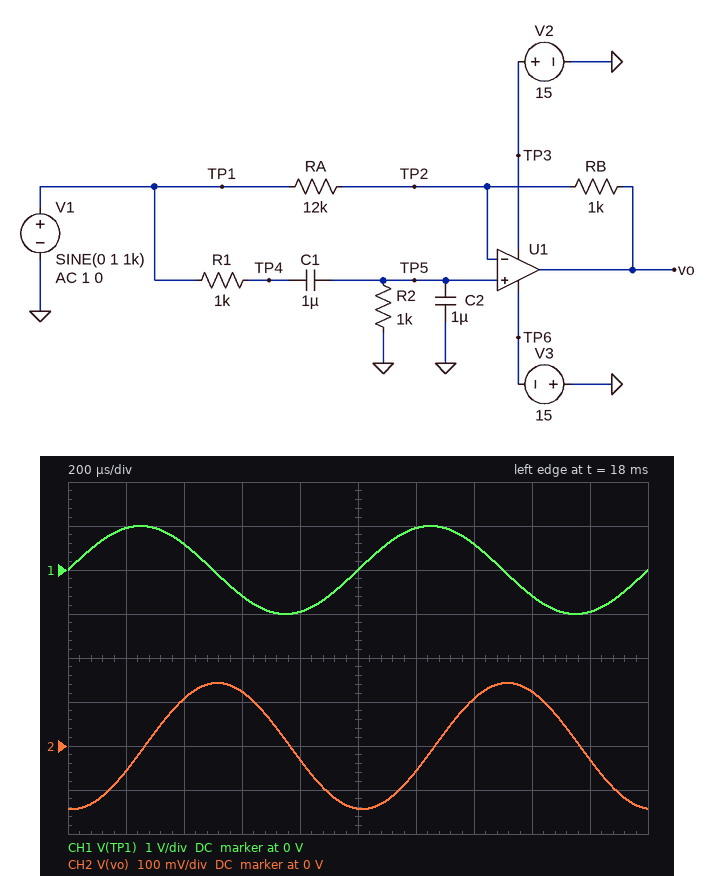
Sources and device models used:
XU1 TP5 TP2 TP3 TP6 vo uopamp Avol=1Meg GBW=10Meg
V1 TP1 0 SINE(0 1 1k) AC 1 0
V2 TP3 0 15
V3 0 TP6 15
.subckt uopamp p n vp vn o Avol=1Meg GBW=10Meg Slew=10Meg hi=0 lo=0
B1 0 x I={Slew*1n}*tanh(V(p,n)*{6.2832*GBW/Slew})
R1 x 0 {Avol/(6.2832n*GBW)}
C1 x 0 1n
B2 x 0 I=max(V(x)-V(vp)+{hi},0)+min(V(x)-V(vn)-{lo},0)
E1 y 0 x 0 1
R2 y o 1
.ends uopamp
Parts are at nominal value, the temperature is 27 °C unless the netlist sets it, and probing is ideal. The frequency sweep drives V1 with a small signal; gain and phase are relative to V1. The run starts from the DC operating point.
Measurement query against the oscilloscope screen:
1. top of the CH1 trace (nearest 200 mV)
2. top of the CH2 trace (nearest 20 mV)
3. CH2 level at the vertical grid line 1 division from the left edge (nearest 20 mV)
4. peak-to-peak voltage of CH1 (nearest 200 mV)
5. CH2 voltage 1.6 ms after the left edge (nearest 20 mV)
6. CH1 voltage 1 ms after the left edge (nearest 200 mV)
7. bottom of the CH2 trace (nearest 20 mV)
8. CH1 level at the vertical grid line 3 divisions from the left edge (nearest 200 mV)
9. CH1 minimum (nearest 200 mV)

1.0 V
140 mV
-60 mV
2.0 V
120 mV
0 V
-140 mV
-600 mV
-1.0 V
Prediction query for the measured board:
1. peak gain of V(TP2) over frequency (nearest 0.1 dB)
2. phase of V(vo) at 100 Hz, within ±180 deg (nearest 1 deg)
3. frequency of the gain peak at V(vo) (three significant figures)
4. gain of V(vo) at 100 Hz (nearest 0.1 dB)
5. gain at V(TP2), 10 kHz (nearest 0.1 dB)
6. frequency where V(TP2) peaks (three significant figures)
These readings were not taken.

-9.5 dB
23 deg
159 Hz
-11.5 dB
-36.0 dB
159 Hz
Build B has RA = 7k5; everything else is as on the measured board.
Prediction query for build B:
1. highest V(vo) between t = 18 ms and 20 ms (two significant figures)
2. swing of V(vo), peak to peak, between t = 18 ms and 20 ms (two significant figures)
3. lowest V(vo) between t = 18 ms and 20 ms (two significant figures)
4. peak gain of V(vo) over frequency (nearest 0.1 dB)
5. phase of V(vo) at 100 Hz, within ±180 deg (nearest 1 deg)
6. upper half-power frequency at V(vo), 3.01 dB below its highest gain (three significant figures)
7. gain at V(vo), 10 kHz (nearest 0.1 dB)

160 mV
320 mV
-160 mV
-12.2 dB
28 deg
783 Hz
-17.5 dB
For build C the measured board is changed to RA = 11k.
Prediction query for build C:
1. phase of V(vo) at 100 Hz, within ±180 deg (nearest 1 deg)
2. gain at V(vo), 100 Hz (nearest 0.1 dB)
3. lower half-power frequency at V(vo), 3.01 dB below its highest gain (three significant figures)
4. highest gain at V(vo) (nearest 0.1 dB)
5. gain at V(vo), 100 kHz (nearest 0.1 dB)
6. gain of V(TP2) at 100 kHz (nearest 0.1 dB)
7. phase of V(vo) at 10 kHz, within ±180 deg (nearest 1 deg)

24 deg
-11.7 dB
43.3 Hz
-11.3 dB
-20.8 dB
-63.3 dB
-169 deg
